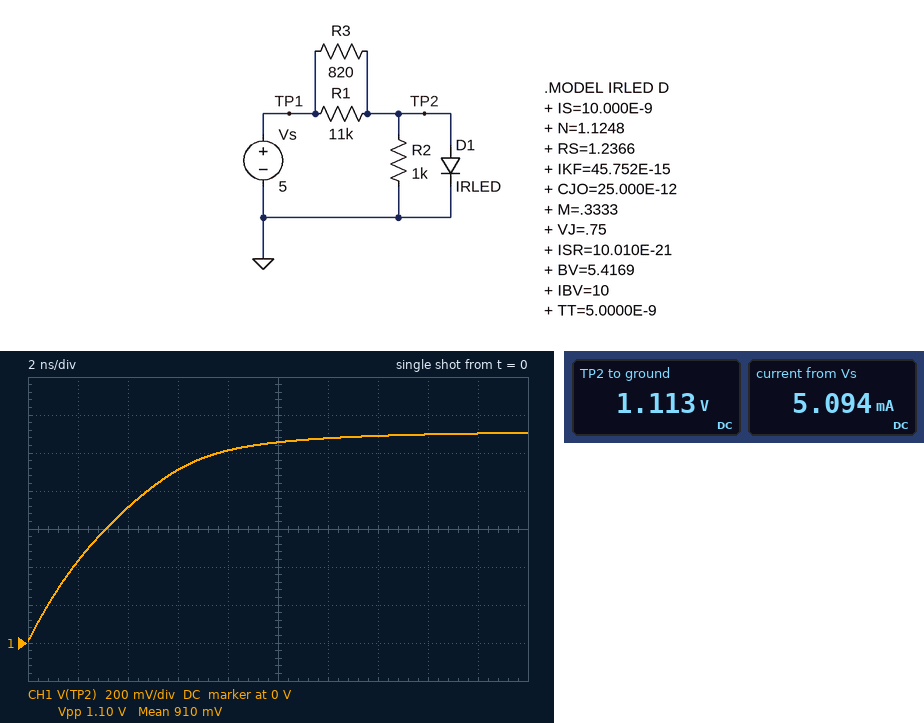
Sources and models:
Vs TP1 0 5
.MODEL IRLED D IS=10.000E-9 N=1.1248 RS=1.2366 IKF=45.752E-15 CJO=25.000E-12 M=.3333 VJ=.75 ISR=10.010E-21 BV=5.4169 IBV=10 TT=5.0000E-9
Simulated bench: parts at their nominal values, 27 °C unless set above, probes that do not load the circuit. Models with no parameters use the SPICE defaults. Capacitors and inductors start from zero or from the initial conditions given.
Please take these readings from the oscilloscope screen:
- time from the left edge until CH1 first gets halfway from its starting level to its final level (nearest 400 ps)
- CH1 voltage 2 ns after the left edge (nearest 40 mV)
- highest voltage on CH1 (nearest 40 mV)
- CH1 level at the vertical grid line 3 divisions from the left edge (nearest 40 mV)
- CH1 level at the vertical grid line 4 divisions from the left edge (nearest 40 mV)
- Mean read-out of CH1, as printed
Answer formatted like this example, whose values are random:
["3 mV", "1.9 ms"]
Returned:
["2.8 ns", "440 mV", "1.12 V", "920 mV", "1.00 V", "910 mV"]
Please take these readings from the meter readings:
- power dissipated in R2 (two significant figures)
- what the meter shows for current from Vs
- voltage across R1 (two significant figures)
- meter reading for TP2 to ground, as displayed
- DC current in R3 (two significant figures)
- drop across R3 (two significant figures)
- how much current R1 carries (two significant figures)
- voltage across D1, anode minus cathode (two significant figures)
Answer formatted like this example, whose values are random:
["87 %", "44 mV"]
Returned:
["1.2 mW", "5.094 mA", "3.9 V", "1.113 V", "4.7 mA", "3.9 V", "350 µA", "1.1 V"]
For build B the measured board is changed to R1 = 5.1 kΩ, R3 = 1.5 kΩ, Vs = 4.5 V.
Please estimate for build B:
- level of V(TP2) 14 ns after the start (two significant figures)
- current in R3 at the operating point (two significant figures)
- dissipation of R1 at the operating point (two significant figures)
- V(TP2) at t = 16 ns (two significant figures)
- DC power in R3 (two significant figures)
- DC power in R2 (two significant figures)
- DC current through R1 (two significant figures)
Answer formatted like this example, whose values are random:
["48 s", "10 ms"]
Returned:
["980 mV", "2.3 mA", "2.3 mW", "1.0 V", "7.9 mW", "1.1 mW", "670 µA"]
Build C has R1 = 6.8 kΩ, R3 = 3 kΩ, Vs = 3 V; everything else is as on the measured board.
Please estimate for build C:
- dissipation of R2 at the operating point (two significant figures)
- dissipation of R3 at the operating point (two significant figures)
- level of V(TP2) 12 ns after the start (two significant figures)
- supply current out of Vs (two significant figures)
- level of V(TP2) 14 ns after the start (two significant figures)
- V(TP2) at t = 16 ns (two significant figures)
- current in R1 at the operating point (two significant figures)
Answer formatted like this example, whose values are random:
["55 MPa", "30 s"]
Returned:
["810 µW", "1.5 mW", "450 mV", "1.0 mA", "490 mV", "530 mV", "310 µA"]
